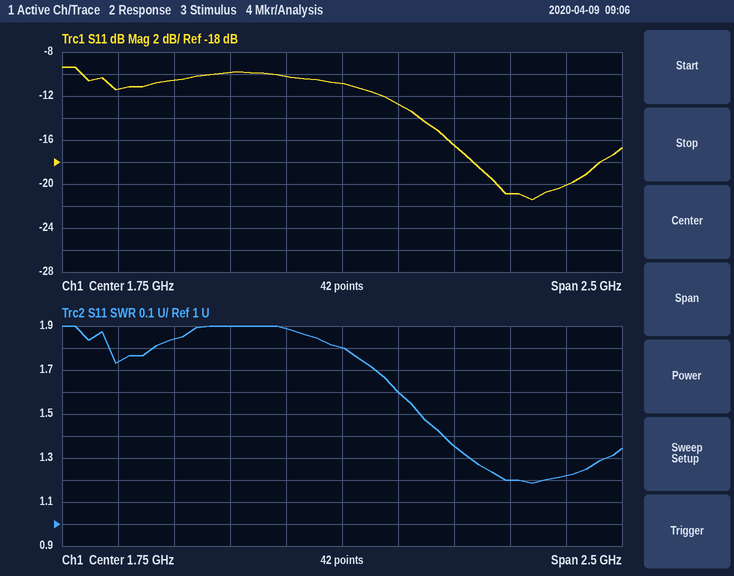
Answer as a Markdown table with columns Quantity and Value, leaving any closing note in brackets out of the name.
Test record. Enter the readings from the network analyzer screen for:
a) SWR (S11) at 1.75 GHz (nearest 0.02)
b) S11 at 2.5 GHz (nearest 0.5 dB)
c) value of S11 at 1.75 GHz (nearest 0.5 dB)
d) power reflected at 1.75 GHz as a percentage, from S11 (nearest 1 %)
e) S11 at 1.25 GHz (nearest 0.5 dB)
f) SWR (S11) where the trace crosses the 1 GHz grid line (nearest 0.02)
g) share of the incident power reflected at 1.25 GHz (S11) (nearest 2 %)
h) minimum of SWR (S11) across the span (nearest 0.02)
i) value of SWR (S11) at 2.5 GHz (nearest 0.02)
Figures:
| Quantity | Value |
|---|---|
| SWR (S11) at 1.75 GHz | 1.80 |
| S11 at 2.5 GHz | -21.0 dB |
| value of S11 at 1.75 GHz | -11.0 dB |
| power reflected at 1.75 GHz as a percentage, from S11 | 8 % |
| S11 at 1.25 GHz | -10.0 dB |
| SWR (S11) where the trace crosses the 1 GHz grid line | 1.84 |
| share of the incident power reflected at 1.25 GHz (S11) | 10 % |
| minimum of SWR (S11) across the span | 1.18 |
| value of SWR (S11) at 2.5 GHz | 1.20 |
